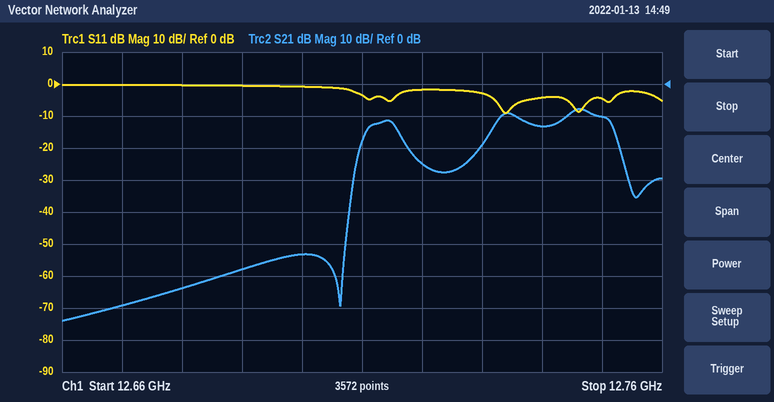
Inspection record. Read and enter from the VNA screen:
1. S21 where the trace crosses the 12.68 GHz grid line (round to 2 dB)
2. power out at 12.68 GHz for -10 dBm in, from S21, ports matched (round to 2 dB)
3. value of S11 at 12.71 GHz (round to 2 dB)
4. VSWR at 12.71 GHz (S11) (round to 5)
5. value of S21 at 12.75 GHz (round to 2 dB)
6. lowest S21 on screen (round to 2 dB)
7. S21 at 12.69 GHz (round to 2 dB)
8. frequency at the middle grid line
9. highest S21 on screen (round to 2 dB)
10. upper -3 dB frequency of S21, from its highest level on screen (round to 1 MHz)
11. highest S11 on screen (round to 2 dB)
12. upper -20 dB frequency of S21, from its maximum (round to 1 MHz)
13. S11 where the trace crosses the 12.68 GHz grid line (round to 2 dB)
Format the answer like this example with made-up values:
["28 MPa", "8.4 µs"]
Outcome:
["-64 dB", "-74 dBm", "-4 dB", "5", "-10 dB", "-74 dB", "-58 dB", "12.71 GHz", "-8 dB", "12.751 GHz", "0 dB", "12.754 GHz", "0 dB"]
